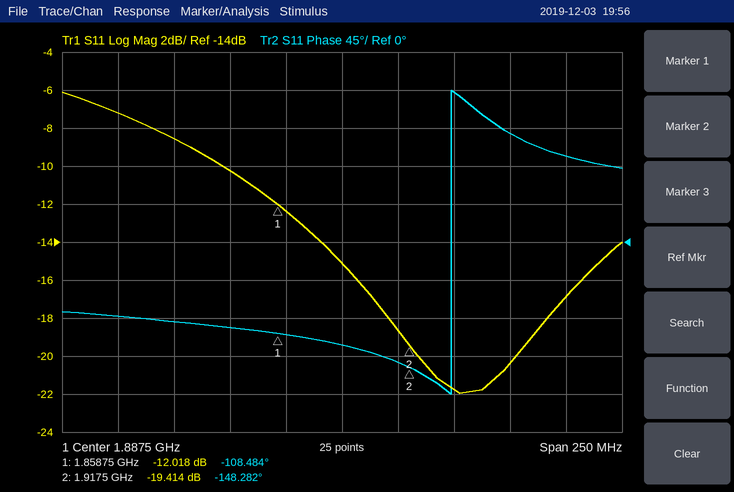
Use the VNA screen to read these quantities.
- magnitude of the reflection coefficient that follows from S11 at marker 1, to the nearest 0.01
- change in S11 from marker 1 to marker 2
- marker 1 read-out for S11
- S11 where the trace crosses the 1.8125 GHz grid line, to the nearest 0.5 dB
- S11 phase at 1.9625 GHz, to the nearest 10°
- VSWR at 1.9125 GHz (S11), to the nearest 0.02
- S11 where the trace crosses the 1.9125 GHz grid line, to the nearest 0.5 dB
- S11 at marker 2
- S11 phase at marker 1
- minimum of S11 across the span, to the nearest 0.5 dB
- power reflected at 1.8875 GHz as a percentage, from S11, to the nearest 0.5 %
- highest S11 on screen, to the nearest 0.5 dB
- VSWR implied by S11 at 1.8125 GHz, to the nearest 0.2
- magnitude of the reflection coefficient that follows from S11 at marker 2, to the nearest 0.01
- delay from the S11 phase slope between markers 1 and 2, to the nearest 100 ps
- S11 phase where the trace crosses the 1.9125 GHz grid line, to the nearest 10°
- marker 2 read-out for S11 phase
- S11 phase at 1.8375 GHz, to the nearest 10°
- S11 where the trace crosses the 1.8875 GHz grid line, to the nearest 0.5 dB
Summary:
0.25
-7.396 dB
-12.018 dB
-8.5 dB
130°
1.26
-18.5 dB
-19.414 dB
-108.484°
-22.0 dB
3.0 %
-6.0 dB
2.2
0.11
1.9 ns
-140°
-148.282°
-100°
-15.0 dB
